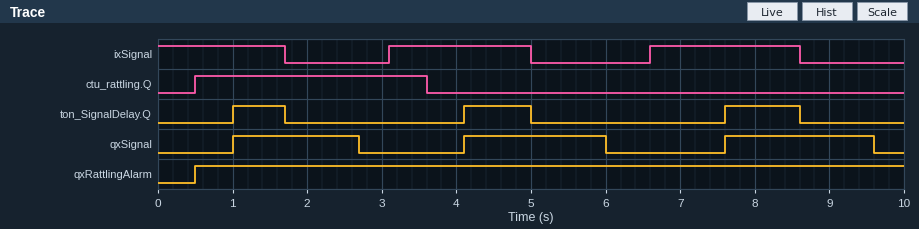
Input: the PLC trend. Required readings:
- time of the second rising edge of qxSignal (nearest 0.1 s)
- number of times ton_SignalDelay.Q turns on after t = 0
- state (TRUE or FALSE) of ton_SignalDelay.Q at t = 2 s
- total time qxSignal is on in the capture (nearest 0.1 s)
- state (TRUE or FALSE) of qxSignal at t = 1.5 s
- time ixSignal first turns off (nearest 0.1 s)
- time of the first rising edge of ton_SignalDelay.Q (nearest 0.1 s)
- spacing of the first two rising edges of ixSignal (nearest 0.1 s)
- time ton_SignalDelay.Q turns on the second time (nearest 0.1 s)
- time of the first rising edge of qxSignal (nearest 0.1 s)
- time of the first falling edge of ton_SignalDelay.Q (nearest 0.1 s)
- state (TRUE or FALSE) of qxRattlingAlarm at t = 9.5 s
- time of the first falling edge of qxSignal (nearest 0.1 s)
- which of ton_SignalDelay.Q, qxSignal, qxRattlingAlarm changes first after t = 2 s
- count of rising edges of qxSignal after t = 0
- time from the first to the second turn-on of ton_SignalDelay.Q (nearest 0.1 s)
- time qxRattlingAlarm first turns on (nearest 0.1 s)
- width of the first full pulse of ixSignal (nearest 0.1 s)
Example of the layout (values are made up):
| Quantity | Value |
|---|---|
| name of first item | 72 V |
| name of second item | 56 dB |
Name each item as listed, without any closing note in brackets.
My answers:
| Quantity | Value |
|---|---|
| time of the second rising edge of qxSignal | 4.1 s |
| number of times ton_SignalDelay.Q turns on after t = 0 | 3 |
| state (TRUE or FALSE) of ton_SignalDelay.Q at t = 2 s | FALSE |
| total time qxSignal is on in the capture | 5.6 s |
| state (TRUE or FALSE) of qxSignal at t = 1.5 s | TRUE |
| time ixSignal first turns off | 1.7 s |
| time of the first rising edge of ton_SignalDelay.Q | 1.0 s |
| spacing of the first two rising edges of ixSignal | 3.5 s |
| time ton_SignalDelay.Q turns on the second time | 4.1 s |
| time of the first rising edge of qxSignal | 1.0 s |
| time of the first falling edge of ton_SignalDelay.Q | 1.7 s |
| state (TRUE or FALSE) of qxRattlingAlarm at t = 9.5 s | TRUE |
| time of the first falling edge of qxSignal | 2.7 s |
| which of ton_SignalDelay.Q, qxSignal, qxRattlingAlarm changes first after t = 2 s | qxSignal |
| count of rising edges of qxSignal after t = 0 | 3 |
| time from the first to the second turn-on of ton_SignalDelay.Q | 3.1 s |
| time qxRattlingAlarm first turns on | 0.5 s |
| width of the first full pulse of ixSignal | 1.9 s |
